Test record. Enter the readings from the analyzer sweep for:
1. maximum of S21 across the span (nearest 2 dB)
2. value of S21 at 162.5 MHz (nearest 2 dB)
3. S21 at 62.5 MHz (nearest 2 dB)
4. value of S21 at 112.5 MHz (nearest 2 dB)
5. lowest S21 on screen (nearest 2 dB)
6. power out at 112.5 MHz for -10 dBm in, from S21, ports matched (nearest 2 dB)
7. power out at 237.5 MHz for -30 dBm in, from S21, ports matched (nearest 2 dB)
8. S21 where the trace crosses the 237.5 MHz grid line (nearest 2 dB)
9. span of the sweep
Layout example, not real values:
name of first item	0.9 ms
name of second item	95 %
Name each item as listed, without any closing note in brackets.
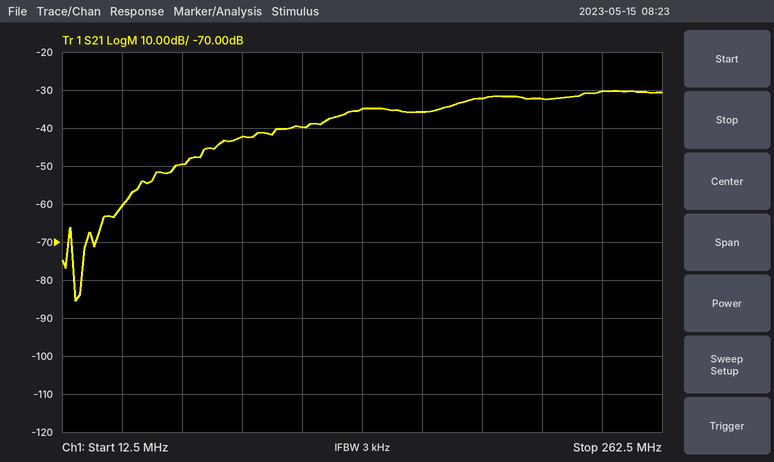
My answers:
maximum of S21 across the span	-30 dB
value of S21 at 162.5 MHz	-36 dB
S21 at 62.5 MHz	-50 dB
value of S21 at 112.5 MHz	-40 dB
lowest S21 on screen	-86 dB
power out at 112.5 MHz for -10 dBm in, from S21, ports matched	-50 dBm
power out at 237.5 MHz for -30 dBm in, from S21, ports matched	-60 dBm
S21 where the trace crosses the 237.5 MHz grid line	-30 dB
span of the sweep	250 MHz
